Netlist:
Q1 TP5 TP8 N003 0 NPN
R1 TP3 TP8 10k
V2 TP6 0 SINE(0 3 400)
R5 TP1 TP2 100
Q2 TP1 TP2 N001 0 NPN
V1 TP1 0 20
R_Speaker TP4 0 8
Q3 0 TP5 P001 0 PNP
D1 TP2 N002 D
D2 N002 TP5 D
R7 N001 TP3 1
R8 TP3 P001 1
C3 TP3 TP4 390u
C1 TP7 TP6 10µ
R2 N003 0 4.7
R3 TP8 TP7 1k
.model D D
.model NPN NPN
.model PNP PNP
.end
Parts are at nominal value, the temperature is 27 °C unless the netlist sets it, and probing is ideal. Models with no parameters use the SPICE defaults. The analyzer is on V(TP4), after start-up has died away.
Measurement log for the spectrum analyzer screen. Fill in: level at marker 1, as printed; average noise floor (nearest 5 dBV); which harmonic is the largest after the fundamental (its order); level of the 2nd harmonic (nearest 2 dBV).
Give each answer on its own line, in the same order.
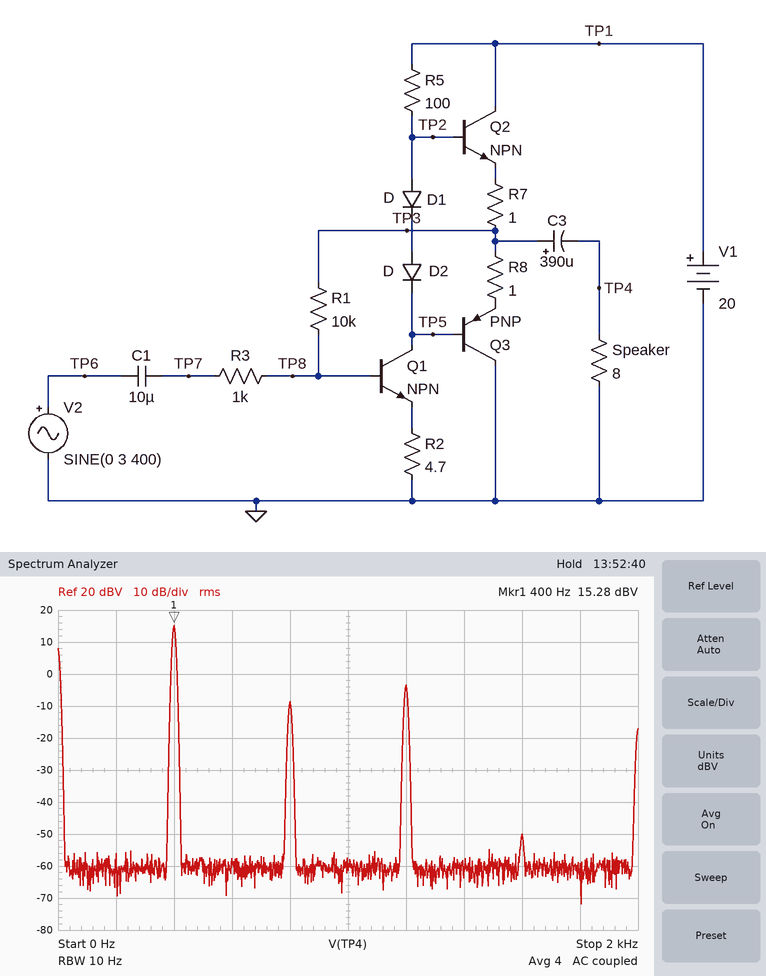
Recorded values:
15.28 dBV
-60 dBV
3
-8 dBV
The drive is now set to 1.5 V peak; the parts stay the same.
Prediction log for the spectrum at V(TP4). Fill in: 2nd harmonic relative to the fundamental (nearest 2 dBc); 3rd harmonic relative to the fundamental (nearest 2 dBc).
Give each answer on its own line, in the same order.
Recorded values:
-48 dBc
-46 dBc
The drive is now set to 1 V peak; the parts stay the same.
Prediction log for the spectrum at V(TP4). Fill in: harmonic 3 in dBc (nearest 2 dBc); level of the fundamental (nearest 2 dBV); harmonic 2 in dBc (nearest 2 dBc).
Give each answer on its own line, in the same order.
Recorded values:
-42 dBc
8 dBV
-52 dBc
